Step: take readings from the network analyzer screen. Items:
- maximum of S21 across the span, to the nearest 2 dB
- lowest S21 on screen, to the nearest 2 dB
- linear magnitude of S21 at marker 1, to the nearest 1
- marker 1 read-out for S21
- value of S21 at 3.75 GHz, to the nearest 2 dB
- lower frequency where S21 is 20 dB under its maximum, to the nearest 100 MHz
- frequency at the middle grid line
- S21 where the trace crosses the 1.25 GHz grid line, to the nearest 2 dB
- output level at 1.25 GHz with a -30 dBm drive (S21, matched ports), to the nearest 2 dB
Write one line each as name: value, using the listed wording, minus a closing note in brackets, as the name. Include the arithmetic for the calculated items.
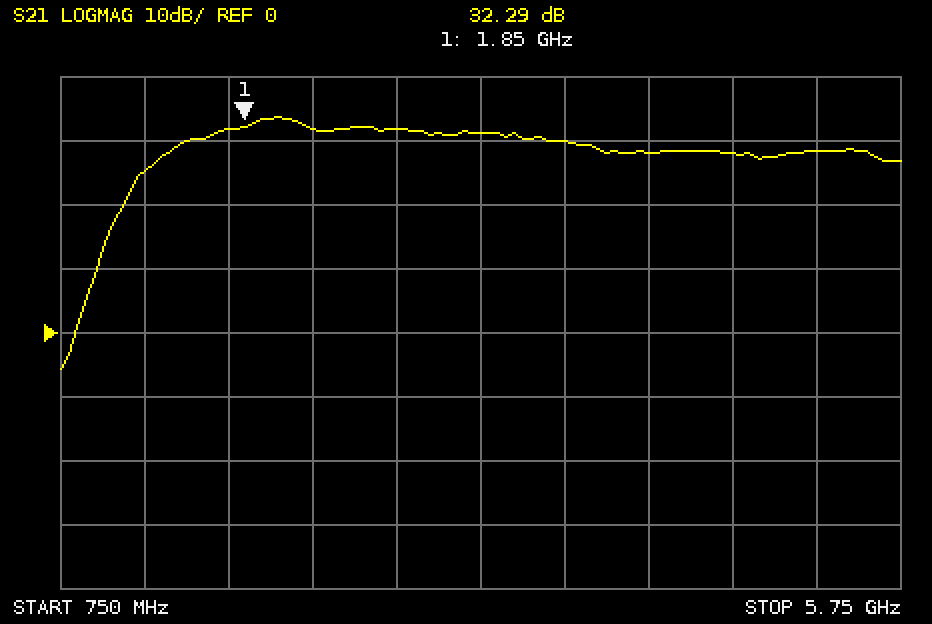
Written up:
maximum of S21 across the span, to the nearest 2 dB: 34 dB
lowest S21 on screen, to the nearest 2 dB: -6 dB
linear magnitude of S21 at marker 1, to the nearest 1: 10^(32.29/20) ≈ 41
marker 1 read-out for S21: 32.29 dB
value of S21 at 3.75 GHz, to the nearest 2 dB: 30 dB
lower frequency where S21 is 20 dB under its maximum, to the nearest 100 MHz: 1.0 GHz
frequency at the middle grid line: 3.25 GHz
S21 where the trace crosses the 1.25 GHz grid line, to the nearest 2 dB: 26 dB
output level at 1.25 GHz with a -30 dBm drive (S21, matched ports), to the nearest 2 dB: -30 dBm + (26 dB) = -4 dBm
